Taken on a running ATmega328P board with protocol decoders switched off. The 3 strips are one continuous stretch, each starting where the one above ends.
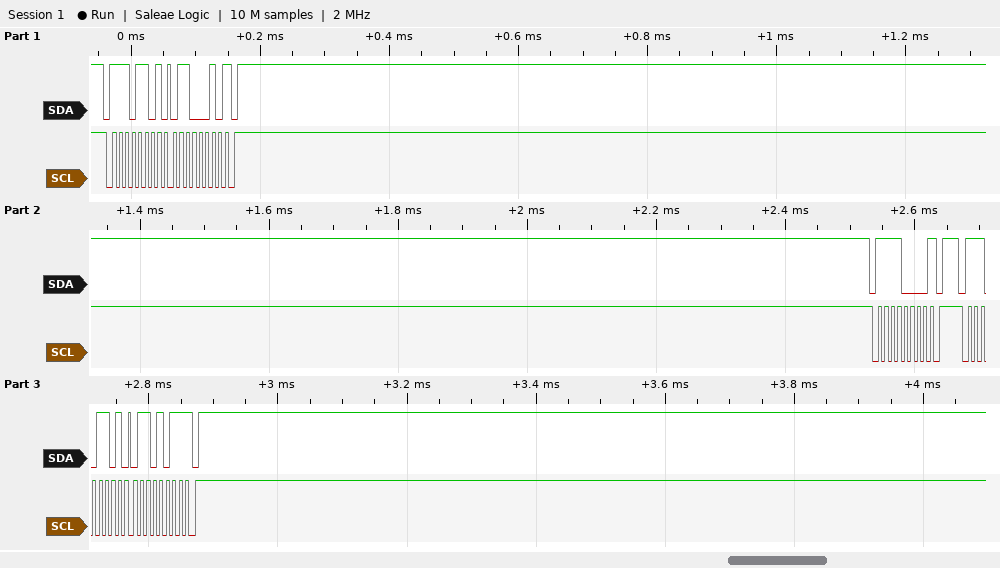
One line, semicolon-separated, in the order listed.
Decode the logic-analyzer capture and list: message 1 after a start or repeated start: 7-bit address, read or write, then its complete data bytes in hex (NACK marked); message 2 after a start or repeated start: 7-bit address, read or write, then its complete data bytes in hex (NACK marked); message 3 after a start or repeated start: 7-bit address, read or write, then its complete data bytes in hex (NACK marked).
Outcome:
0x76 read: 62 NACK; 0x78 write NACK; 0x76 read: 6B NACK
